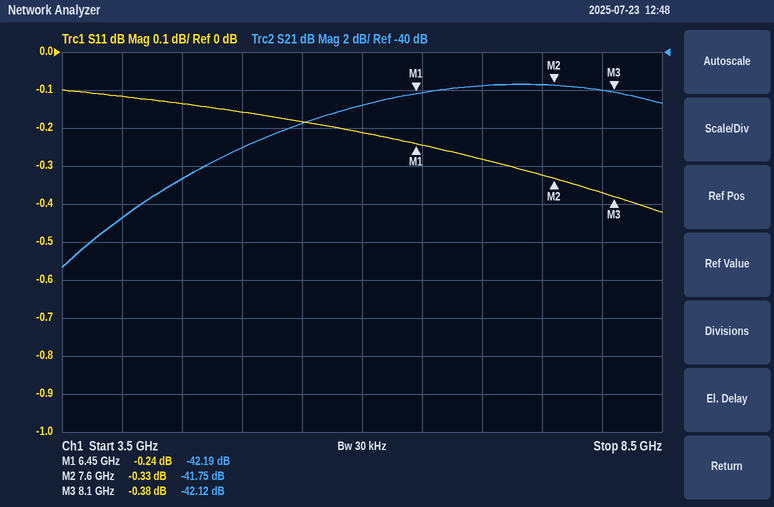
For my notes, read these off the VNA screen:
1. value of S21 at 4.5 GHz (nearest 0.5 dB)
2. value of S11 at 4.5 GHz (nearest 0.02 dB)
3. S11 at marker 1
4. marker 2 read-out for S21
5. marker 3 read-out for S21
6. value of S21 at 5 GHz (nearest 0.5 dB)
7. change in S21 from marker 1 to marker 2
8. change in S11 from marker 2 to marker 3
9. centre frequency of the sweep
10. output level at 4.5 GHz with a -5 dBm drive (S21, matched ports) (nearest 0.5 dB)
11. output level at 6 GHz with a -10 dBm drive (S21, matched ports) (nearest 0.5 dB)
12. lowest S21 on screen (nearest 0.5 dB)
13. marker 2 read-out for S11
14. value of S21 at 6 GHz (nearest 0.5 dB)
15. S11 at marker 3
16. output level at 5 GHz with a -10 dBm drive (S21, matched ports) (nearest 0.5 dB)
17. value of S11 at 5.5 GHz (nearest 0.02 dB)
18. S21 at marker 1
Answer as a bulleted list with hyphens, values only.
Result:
- -46.5 dB
- -0.14 dB
- -0.24 dB
- -41.75 dB
- -42.12 dB
- -45.0 dB
- 0.44 dB
- -0.05 dB
- 6 GHz
- -51.5 dBm
- -53.0 dBm
- -51.5 dB
- -0.33 dB
- -43.0 dB
- -0.38 dB
- -55.0 dBm
- -0.18 dB
- -42.19 dB
